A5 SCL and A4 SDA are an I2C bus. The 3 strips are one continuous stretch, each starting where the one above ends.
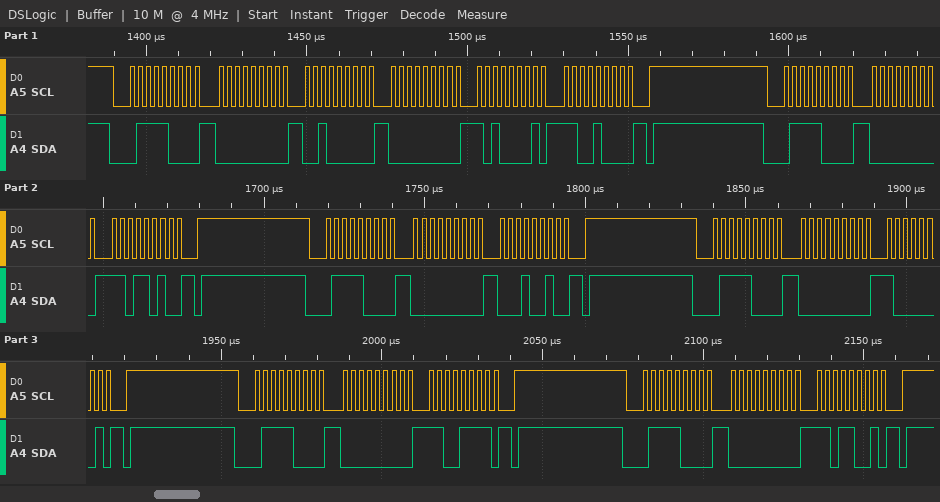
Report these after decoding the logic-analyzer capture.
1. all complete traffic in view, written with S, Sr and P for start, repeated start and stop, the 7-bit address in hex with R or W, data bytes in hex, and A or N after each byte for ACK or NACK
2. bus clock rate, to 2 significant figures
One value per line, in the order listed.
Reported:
S 3CW A 00 A 20 A 00 A A1 A C8 A P S 3CW A 00 A DA A P S 3CW A 00 A 12 A P S 3CW A 00 A 81 A P S 3CW A 00 A CF A P S 3CW A 00 A D9 A P
400 kHz
